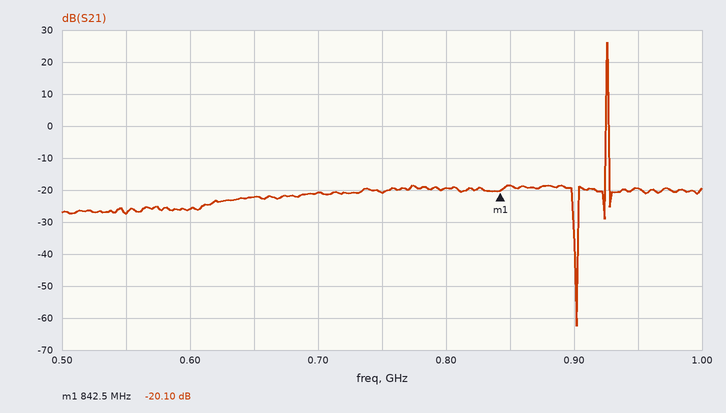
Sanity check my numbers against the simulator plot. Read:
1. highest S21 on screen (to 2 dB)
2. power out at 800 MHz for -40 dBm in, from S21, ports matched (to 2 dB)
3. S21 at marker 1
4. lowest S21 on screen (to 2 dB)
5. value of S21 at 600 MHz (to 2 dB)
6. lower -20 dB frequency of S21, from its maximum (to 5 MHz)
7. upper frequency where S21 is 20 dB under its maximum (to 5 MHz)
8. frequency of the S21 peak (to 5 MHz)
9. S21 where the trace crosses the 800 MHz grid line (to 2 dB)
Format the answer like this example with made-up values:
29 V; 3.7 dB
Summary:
26 dB; -60 dBm; -20.10 dB; -62 dB; -26 dB; 925 MHz; 925 MHz; 925 MHz; -20 dB
